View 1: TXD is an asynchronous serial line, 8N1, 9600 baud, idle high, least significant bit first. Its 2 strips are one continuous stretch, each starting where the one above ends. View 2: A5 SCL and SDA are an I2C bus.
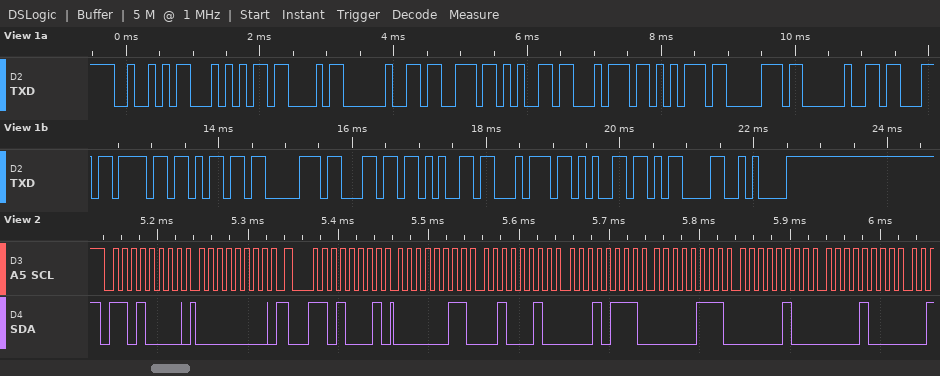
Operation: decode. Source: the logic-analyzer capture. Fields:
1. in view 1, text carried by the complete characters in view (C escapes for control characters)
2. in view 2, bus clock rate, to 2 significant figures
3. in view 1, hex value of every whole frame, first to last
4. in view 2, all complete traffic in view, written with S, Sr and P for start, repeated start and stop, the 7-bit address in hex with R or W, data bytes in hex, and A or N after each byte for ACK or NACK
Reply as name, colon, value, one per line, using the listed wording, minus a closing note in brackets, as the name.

in view 1, text carried by the complete characters in view: "RTC setup complete\r\n"
in view 2, bus clock rate, to 2 significant figures: 100 kHz
in view 1, hex value of every whole frame, first to last: 52 54 43 20 73 65 74 75 70 20 63 6F 6D 70 6C 65 74 65 0D 0A
in view 2, all complete traffic in view, written with S, Sr and P for start, repeated start and stop, the 7-bit address in hex with R or W, data bytes in hex, and A or N after each byte for ACK or NACK: S 68W A 00 A Sr 68R A 03 A 22 A 17 A 07 A 04 A 08 A
